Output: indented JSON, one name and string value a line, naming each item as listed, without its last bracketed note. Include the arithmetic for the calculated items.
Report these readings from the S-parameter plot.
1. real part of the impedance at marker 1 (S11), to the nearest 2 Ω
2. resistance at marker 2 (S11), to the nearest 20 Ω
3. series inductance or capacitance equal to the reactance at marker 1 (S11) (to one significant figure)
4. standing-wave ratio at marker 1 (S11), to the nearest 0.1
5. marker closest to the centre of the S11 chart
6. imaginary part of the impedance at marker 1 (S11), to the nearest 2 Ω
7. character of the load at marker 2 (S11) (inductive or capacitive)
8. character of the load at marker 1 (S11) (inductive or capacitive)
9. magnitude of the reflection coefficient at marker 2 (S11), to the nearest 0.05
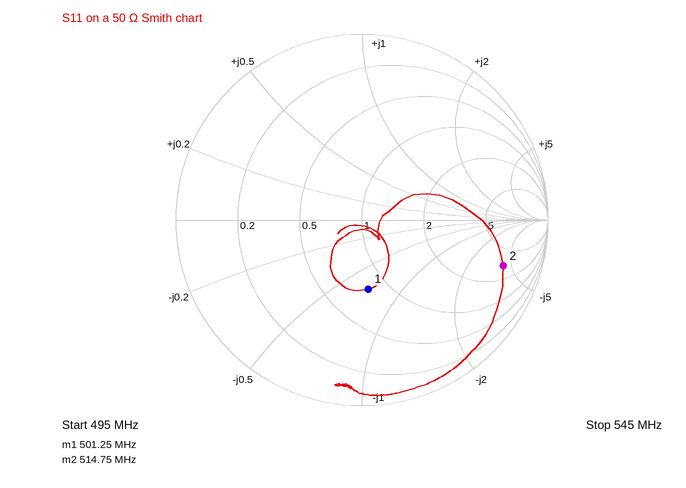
{
  "real part of the impedance at marker 1 (S11), to the nearest 2 Ω": "40 Ω",
  "resistance at marker 2 (S11), to the nearest 20 Ω": "160 Ω",
  "series inductance or capacitance equal to the reactance at marker 1 (S11)": "C = 1/(2π × 501.25 MHz × 34 Ω) ≈ 9 pF",
  "standing-wave ratio at marker 1 (S11), to the nearest 0.1": "2.2",
  "marker closest to the centre of the S11 chart": "marker 1",
  "imaginary part of the impedance at marker 1 (S11), to the nearest 2 Ω": "-34 Ω",
  "character of the load at marker 2 (S11)": "capacitive",
  "character of the load at marker 1 (S11)": "capacitive",
  "magnitude of the reflection coefficient at marker 2 (S11), to the nearest 0.05": "0.80"
}
